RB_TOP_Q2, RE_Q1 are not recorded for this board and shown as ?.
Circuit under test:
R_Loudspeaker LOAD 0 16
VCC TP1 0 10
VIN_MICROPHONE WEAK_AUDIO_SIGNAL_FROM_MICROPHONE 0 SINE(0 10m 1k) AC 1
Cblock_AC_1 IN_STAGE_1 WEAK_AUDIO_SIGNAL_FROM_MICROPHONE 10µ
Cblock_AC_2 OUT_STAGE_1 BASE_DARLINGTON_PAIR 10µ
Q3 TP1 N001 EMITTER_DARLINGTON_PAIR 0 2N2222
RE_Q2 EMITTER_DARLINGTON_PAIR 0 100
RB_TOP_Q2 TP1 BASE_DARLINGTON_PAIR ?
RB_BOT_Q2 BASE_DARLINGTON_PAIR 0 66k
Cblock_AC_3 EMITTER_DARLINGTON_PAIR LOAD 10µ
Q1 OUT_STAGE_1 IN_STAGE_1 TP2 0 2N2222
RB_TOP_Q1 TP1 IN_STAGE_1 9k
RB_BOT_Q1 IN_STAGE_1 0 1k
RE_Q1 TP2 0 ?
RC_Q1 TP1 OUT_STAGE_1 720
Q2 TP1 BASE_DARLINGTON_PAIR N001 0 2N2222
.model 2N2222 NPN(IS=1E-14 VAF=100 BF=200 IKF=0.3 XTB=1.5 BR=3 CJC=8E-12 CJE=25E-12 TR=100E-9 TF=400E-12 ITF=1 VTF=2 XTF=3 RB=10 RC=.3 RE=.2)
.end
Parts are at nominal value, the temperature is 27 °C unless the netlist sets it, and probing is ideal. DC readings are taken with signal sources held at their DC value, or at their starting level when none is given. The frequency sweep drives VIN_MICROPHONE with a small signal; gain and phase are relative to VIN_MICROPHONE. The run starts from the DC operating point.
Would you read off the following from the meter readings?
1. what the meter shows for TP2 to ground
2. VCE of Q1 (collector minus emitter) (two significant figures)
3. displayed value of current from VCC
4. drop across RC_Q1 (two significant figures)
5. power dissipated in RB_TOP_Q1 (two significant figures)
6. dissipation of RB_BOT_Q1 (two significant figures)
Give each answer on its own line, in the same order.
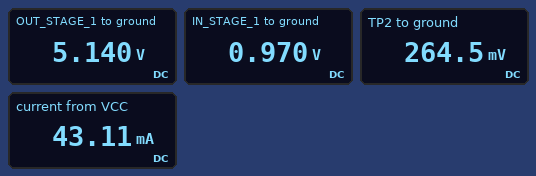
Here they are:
264.5 mV
4.9 V
43.11 mA
4.9 V
9.1 mW
940 µW
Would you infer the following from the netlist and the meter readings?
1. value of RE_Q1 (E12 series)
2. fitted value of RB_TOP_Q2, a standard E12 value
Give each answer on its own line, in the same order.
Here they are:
39 Ω
68 kΩ
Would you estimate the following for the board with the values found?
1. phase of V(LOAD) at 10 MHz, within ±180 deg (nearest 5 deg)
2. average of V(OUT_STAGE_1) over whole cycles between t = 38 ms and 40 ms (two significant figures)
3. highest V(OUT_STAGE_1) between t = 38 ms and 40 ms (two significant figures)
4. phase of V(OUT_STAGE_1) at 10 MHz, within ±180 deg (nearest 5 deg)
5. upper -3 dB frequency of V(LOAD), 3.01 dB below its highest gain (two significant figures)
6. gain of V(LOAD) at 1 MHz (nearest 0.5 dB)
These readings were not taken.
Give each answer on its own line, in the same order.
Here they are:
120 deg
5.1 V
5.3 V
130 deg
13 MHz
23.0 dB
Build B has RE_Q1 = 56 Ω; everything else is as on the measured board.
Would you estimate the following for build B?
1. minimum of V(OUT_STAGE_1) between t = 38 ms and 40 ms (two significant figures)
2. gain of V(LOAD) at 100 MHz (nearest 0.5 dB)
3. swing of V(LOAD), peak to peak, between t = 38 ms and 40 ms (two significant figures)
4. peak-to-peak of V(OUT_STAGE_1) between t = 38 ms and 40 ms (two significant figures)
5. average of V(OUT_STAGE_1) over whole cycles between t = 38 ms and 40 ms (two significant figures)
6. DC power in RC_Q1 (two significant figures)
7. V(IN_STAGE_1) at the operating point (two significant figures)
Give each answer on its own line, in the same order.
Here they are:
6.3 V
-6.0 dB
150 mV
230 mV
6.4 V
18 mW
980 mV
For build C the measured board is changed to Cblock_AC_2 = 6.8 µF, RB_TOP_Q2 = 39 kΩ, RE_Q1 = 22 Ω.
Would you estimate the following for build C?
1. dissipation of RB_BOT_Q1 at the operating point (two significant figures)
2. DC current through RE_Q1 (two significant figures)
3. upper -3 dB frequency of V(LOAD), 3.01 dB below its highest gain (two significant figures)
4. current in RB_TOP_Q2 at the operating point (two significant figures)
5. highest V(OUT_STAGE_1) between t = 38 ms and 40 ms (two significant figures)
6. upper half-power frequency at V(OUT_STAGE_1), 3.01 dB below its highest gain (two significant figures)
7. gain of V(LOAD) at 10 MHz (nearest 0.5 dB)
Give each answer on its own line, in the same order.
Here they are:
910 µW
11 mA
14 MHz
96 µA
2.7 V
15 MHz
27.0 dB
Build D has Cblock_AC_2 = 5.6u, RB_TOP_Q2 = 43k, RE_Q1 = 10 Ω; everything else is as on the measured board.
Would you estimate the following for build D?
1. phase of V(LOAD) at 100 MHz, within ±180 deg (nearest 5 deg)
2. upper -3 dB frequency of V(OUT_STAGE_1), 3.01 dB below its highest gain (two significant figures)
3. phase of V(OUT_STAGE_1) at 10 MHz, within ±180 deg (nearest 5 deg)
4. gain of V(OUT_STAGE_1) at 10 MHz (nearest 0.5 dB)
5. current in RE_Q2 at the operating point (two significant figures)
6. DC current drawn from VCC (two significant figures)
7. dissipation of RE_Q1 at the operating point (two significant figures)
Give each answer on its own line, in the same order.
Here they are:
-15 deg
800 kHz
55 deg
-0.5 dB
46 mA
61 mA
1.9 mW
